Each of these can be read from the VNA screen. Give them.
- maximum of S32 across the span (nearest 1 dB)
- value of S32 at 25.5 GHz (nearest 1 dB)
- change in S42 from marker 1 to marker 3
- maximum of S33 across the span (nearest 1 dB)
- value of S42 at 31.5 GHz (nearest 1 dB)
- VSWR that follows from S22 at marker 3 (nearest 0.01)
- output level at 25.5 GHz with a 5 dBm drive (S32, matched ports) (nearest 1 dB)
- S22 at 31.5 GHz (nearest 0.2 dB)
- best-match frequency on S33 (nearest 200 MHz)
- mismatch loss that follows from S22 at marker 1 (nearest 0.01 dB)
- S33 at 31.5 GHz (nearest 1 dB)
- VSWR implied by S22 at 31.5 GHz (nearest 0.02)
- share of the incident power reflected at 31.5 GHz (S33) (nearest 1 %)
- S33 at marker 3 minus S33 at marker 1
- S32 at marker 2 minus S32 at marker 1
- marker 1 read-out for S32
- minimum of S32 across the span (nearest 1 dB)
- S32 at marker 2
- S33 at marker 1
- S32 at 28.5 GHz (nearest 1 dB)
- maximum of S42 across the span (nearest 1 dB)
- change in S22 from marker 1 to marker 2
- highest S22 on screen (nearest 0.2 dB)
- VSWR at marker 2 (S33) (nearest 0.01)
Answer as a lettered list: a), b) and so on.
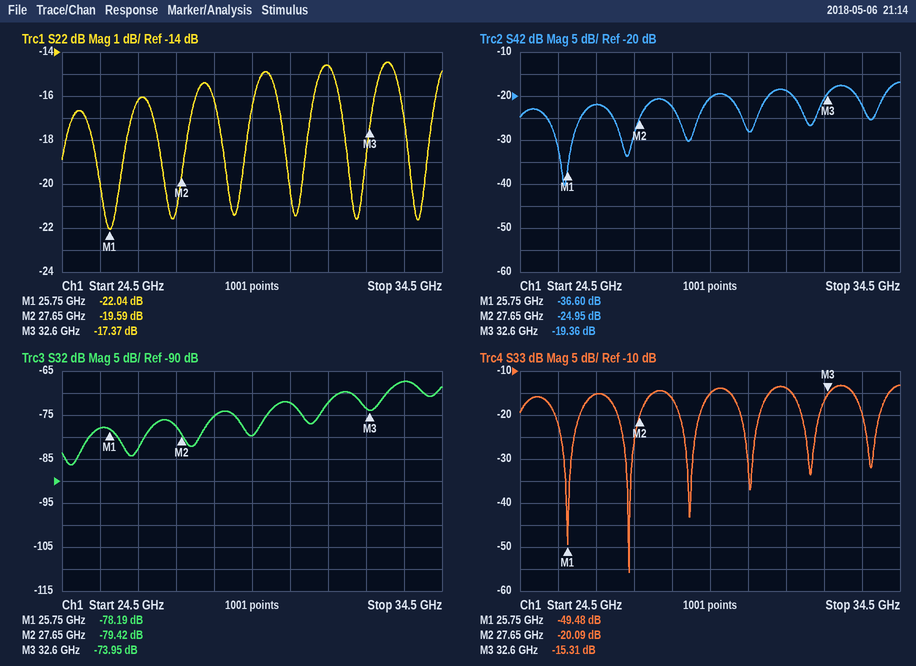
a) -67 dB
b) -78 dB
c) 17.24 dB
d) -13 dB
e) -19 dB
f) 1.31
g) -73 dBm
h) -14.6 dB
i) 27.4 GHz
j) 0.03 dB
k) -14 dB
l) 1.46
m) 4 %
n) 34.17 dB
o) -1.23 dB
p) -78.19 dB
q) -86 dB
r) -79.42 dB
s) -49.48 dB
t) -75 dB
u) -17 dB
v) 2.45 dB
w) -14.4 dB
x) 1.22
